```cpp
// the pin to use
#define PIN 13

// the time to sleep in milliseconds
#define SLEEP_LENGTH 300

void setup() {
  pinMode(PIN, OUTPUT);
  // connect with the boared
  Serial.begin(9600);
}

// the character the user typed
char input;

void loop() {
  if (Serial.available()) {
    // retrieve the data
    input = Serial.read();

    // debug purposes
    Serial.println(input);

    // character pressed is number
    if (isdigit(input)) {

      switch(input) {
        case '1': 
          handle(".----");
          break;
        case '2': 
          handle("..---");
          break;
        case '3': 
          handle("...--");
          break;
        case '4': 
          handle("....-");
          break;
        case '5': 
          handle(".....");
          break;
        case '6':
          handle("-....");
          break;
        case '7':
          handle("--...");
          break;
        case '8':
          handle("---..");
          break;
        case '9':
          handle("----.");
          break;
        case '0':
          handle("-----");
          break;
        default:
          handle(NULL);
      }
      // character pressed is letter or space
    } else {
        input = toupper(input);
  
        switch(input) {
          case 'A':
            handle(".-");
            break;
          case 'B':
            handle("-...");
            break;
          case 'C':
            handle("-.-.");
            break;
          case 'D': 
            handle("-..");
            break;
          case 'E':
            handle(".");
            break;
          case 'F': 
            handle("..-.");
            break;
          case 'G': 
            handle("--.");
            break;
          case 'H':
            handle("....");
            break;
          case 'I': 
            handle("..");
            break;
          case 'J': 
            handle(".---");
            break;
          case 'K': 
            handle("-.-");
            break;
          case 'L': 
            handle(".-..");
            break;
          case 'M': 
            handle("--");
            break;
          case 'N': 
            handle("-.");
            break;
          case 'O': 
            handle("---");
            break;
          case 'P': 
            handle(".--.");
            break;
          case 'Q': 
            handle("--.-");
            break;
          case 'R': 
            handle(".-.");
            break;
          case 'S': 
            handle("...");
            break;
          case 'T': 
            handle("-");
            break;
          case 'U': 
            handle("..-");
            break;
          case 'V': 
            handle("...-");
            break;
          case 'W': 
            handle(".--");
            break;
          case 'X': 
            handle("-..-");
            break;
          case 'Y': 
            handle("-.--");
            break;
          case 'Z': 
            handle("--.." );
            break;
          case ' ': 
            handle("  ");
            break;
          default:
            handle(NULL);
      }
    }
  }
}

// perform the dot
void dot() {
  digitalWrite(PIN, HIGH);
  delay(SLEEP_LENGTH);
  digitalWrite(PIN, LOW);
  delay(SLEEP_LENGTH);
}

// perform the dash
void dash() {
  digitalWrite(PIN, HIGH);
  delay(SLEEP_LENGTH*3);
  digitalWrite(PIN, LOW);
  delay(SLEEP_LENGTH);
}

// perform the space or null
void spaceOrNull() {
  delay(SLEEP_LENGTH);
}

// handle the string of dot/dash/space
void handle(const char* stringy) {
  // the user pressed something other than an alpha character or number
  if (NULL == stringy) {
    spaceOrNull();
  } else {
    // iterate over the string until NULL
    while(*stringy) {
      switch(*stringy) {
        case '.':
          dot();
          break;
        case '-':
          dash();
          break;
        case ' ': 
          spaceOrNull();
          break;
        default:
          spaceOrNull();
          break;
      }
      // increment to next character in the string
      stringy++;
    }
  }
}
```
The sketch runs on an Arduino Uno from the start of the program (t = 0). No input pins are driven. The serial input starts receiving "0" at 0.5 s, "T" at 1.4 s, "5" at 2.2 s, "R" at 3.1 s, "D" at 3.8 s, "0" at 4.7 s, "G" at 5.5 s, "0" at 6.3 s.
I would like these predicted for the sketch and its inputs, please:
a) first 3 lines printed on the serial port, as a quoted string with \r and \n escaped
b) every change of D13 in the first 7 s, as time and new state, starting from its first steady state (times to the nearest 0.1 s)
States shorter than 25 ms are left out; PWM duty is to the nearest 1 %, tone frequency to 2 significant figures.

"0\r\nT\r\n5\r\n"
0 s low; 0.5 s high; 1.4 s low; 1.7 s high; 2.6 s low; 2.9 s high; 3.8 s low; 4.1 s high; 5 s low; 5.3 s high; 6.2 s low; 6.5 s high
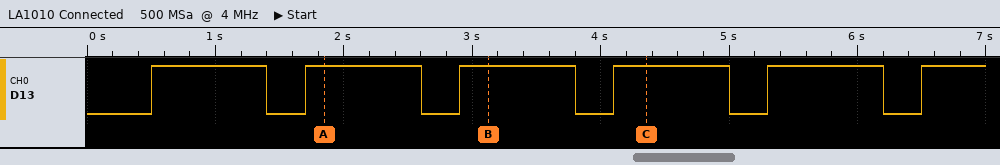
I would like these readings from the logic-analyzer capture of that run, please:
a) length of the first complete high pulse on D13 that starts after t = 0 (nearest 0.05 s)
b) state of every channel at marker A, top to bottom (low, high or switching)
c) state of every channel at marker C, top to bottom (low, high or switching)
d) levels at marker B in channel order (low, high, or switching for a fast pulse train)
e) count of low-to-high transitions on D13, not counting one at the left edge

0.90 s
D13 high
D13 high
D13 high
6
